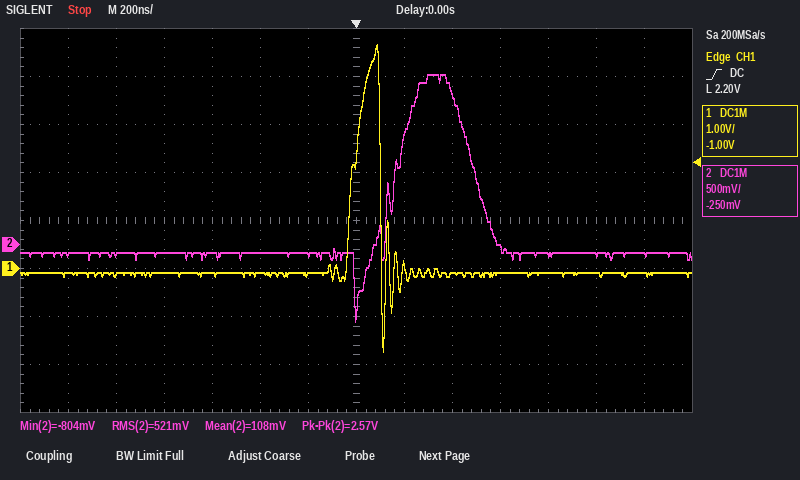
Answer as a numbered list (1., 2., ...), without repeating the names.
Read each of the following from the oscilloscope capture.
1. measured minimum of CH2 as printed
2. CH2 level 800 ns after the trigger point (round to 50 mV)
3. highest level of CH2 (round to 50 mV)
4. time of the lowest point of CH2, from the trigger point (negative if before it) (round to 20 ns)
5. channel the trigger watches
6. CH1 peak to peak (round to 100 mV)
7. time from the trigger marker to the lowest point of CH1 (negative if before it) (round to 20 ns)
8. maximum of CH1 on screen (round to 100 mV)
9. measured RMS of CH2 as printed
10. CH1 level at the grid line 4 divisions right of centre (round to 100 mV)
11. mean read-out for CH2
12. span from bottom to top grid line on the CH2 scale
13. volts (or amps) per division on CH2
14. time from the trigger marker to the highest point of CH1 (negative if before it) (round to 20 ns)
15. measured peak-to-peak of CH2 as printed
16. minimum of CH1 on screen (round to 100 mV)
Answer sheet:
1. -804 mV
2. -100 mV
3. 1.75 V
4. 0 ns
5. CH1
6. 6.4 V
7. +120 ns
8. 4.7 V
9. 521 mV
10. -100 mV
11. 108 mV
12. 4 V
13. 500 mV
14. +80 ns
15. 2.57 V
16. -1.7 V
